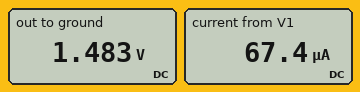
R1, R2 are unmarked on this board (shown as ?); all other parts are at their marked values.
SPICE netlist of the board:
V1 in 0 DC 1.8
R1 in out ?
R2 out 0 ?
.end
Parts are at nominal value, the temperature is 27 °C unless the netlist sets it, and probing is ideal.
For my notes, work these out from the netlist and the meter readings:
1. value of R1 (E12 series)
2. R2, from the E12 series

4.7 kΩ
22 kΩ
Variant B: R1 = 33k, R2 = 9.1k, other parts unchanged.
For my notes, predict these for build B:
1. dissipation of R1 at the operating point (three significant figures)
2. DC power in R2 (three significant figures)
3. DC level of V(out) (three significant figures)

60.3 µW
16.6 µW
389 mV
